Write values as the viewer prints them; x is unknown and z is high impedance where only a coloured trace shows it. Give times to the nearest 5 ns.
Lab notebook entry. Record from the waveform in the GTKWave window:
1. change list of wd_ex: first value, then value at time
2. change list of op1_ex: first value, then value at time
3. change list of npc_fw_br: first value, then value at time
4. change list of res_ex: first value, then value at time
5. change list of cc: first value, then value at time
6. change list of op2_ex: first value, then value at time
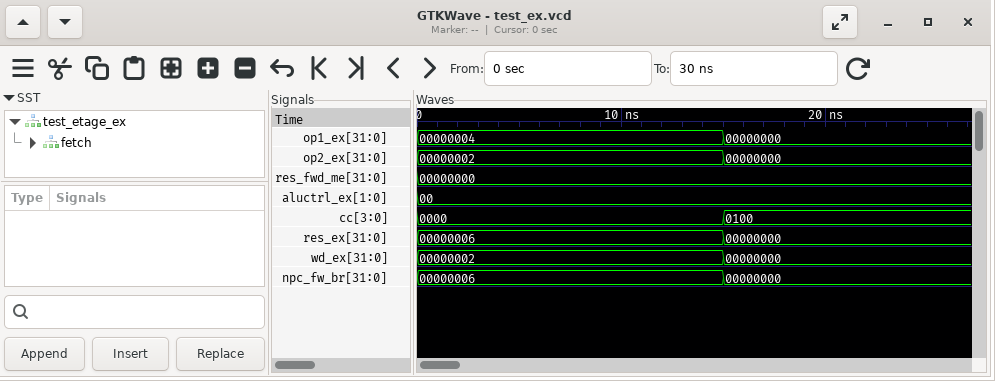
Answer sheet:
00000002, 00000000 at 15 ns
00000004, 00000000 at 15 ns
00000006, 00000000 at 15 ns
00000006, 00000000 at 15 ns
0000, 0100 at 15 ns
00000002, 00000000 at 15 ns
